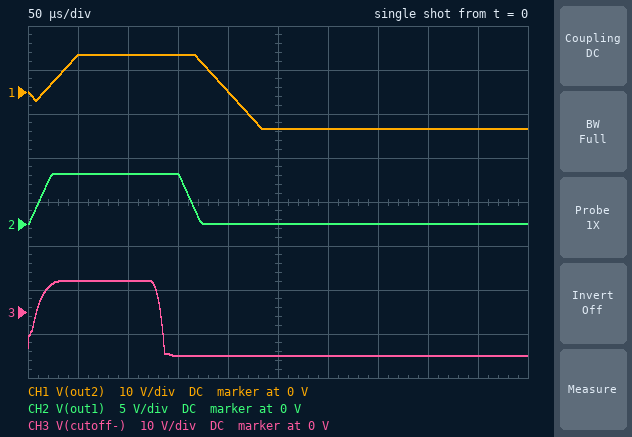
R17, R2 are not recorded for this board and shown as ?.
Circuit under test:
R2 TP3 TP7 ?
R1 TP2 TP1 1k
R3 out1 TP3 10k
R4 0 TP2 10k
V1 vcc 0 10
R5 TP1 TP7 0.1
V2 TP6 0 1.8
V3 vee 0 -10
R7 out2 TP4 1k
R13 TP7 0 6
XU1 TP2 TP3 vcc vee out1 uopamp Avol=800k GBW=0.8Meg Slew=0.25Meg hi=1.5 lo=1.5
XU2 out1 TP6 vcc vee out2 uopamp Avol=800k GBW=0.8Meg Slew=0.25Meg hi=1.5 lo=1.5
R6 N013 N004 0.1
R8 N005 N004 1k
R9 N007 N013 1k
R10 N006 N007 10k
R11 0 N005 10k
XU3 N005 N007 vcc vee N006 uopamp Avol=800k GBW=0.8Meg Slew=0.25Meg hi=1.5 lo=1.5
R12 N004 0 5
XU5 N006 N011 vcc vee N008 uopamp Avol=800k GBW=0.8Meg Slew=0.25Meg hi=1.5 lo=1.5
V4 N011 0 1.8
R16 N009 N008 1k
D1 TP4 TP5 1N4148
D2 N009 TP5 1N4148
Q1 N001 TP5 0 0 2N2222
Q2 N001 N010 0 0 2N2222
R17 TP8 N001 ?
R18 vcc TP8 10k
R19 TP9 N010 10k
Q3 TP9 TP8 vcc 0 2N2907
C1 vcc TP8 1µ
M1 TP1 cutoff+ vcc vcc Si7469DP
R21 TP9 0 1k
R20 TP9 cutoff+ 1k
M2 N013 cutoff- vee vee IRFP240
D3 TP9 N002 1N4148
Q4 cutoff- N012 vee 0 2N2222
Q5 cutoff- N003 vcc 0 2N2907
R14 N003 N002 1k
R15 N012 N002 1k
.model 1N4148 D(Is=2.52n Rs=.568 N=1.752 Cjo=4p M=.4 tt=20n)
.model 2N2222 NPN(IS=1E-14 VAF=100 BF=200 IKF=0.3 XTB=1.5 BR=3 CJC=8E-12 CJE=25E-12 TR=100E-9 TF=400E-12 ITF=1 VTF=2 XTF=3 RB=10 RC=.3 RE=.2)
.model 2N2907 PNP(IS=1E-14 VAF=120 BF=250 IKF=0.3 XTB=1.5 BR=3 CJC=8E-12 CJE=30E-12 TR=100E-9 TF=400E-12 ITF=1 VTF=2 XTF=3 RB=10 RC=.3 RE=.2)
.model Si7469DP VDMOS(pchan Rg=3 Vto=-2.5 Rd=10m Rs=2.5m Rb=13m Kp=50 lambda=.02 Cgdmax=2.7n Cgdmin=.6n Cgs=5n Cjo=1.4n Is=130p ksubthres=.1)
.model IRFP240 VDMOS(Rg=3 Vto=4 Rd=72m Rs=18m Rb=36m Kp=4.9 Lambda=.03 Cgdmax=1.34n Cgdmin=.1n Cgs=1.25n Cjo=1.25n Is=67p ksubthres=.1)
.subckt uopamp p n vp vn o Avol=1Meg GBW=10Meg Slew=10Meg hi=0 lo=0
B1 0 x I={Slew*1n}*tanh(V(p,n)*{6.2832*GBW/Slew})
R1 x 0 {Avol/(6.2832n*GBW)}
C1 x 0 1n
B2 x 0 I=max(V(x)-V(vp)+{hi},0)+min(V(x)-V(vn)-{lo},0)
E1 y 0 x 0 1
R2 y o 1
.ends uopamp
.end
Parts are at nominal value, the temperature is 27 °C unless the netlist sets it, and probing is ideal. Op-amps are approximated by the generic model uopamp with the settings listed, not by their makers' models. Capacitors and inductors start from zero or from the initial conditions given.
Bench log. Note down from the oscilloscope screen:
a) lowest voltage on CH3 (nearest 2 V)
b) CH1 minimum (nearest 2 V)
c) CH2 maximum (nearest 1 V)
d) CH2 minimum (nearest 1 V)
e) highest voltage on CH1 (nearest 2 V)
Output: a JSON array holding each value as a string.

["-10 V", "-8 V", "6 V", "0 V", "8 V"]
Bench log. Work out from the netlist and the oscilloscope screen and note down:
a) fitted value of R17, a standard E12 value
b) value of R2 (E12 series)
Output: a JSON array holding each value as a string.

["1.8 kΩ", "2.2 kΩ"]
